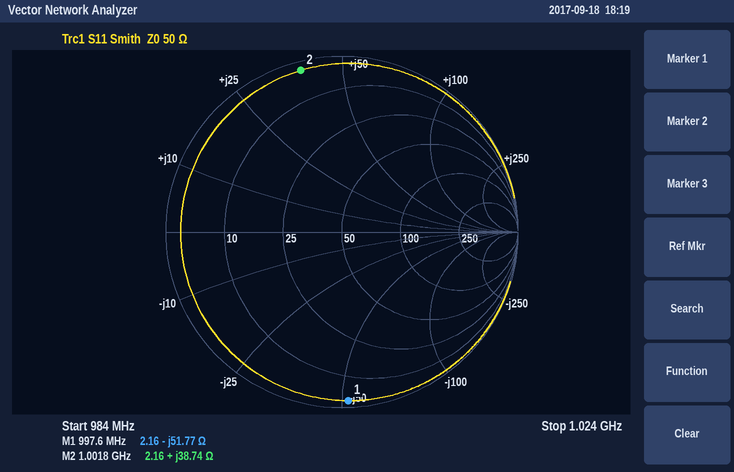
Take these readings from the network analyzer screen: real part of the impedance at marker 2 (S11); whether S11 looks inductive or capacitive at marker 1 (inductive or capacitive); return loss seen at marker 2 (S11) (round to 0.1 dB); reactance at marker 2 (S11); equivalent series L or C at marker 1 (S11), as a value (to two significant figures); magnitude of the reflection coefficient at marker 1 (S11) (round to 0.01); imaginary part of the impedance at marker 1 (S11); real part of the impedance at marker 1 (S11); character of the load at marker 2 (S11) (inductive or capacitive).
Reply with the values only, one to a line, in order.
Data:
2.16 Ω
capacitive
0.5 dB
+38.74 Ω
3.1 pF
0.96
-51.77 Ω
2.16 Ω
inductive
